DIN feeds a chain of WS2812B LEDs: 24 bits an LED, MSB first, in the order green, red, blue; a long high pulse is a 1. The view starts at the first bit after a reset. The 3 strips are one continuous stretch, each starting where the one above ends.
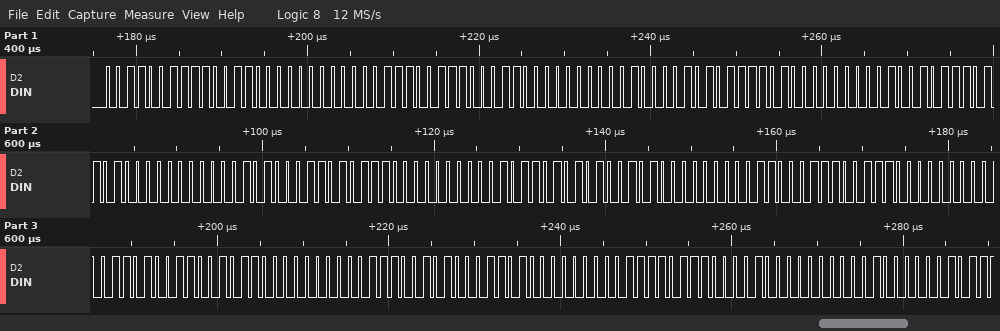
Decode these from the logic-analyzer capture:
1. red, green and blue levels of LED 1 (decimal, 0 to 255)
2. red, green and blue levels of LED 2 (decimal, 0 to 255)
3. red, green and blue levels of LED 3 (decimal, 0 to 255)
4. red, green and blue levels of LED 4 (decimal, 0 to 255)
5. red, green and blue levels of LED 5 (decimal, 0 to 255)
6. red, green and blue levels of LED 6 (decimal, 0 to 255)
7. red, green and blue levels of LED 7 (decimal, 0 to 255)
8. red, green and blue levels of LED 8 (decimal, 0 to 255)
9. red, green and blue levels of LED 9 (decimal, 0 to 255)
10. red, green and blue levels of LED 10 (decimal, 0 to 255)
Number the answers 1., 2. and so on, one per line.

1. 204, 51, 0
2. 198, 57, 0
3. 189, 66, 0
4. 180, 75, 0
5. 174, 81, 0
6. 165, 90, 0
7. 156, 99, 0
8. 150, 105, 0
9. 141, 114, 0
10. 132, 123, 0
